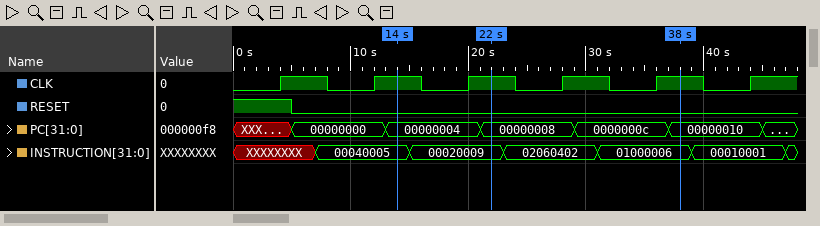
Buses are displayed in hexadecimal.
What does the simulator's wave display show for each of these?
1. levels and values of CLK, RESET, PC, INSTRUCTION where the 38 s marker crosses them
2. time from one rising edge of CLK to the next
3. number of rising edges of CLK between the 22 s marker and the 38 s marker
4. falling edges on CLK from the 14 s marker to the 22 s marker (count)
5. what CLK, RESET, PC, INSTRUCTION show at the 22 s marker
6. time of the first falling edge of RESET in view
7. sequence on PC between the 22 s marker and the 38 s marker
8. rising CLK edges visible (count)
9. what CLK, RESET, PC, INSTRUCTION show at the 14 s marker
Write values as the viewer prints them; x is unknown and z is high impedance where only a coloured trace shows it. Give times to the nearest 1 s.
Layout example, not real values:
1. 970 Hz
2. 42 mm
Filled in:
1. CLK=1, RESET=0, PC=00000010, INSTRUCTION=01000006
2. 8 s
3. 2
4. 1
5. CLK=1, RESET=0, PC=00000008, INSTRUCTION=00020009
6. 5 s
7. 00000008, 0000000c, 00000010
8. 6
9. CLK=1, RESET=0, PC=00000004, INSTRUCTION=00040005
